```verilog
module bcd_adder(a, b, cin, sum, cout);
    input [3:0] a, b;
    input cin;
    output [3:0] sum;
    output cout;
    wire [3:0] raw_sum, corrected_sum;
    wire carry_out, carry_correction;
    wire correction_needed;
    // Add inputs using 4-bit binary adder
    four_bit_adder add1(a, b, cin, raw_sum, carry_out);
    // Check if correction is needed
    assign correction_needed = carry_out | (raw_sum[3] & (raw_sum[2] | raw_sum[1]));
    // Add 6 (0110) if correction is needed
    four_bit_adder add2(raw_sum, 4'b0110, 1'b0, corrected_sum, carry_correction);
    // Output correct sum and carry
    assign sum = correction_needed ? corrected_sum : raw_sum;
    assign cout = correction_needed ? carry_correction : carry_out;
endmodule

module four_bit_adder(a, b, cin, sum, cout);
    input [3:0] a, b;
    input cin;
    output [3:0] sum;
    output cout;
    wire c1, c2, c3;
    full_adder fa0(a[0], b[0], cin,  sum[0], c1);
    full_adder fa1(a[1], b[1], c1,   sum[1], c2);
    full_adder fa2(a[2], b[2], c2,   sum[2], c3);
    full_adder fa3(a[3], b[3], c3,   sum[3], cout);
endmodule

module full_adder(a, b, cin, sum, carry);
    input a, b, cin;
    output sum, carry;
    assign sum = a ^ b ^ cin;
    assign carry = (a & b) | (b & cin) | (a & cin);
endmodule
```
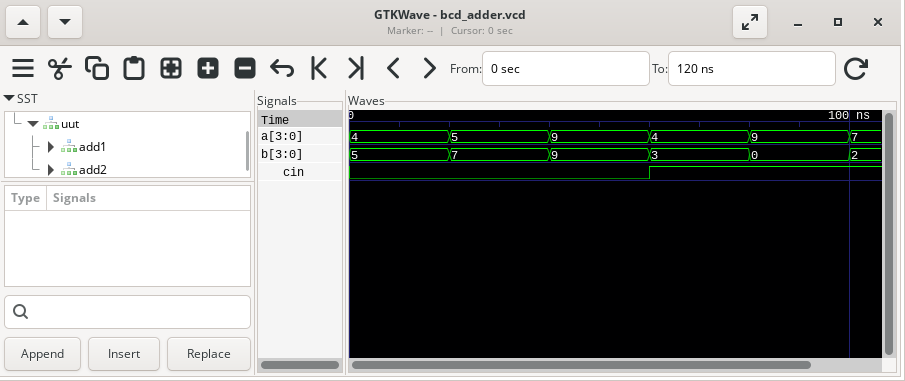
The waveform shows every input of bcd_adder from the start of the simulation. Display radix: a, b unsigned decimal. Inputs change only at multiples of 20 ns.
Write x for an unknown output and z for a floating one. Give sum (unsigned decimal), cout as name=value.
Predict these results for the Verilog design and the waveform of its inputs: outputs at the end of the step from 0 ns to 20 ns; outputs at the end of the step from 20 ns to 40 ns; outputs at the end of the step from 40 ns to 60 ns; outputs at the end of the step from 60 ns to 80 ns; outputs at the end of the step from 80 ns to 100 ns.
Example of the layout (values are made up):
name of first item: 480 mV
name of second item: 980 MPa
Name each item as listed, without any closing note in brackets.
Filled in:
outputs at the end of the step from 0 ns to 20 ns: sum=9, cout=0
outputs at the end of the step from 20 ns to 40 ns: sum=2, cout=1
outputs at the end of the step from 40 ns to 60 ns: sum=8, cout=0
outputs at the end of the step from 60 ns to 80 ns: sum=8, cout=0
outputs at the end of the step from 80 ns to 100 ns: sum=0, cout=1
